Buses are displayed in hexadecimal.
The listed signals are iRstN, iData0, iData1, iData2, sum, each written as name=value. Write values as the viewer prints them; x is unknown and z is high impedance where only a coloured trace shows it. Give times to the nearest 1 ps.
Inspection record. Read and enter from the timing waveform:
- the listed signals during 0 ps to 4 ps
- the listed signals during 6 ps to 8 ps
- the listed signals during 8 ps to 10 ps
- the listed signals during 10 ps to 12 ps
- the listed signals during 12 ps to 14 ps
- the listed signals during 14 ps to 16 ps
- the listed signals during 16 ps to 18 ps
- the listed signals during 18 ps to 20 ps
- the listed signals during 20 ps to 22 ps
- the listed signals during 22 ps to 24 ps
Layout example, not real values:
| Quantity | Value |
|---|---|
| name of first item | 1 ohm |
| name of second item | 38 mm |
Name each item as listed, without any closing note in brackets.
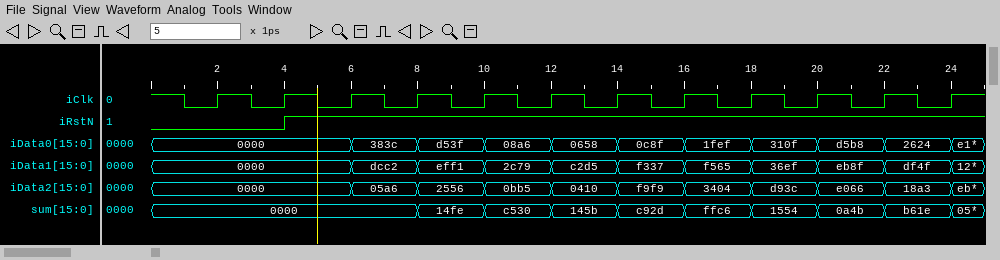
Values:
| Quantity | Value |
|---|---|
| the listed signals during 0 ps to 4 ps | iRstN=0, iData0=0000, iData1=0000, iData2=0000, sum=0000 |
| the listed signals during 6 ps to 8 ps | iRstN=1, iData0=383c, iData1=dcc2, iData2=05a6, sum=0000 |
| the listed signals during 8 ps to 10 ps | iRstN=1, iData0=d53f, iData1=eff1, iData2=2556, sum=14fe |
| the listed signals during 10 ps to 12 ps | iRstN=1, iData0=08a6, iData1=2c79, iData2=0bb5, sum=c530 |
| the listed signals during 12 ps to 14 ps | iRstN=1, iData0=0658, iData1=c2d5, iData2=0410, sum=145b |
| the listed signals during 14 ps to 16 ps | iRstN=1, iData0=0c8f, iData1=f337, iData2=f9f9, sum=c92d |
| the listed signals during 16 ps to 18 ps | iRstN=1, iData0=1fef, iData1=f565, iData2=3404, sum=ffc6 |
| the listed signals during 18 ps to 20 ps | iRstN=1, iData0=310f, iData1=36ef, iData2=d93c, sum=1554 |
| the listed signals during 20 ps to 22 ps | iRstN=1, iData0=d5b8, iData1=eb8f, iData2=e066, sum=0a4b |
| the listed signals during 22 ps to 24 ps | iRstN=1, iData0=2624, iData1=df4f, iData2=18a3, sum=b61e |
